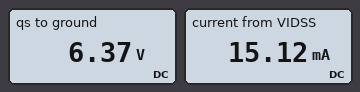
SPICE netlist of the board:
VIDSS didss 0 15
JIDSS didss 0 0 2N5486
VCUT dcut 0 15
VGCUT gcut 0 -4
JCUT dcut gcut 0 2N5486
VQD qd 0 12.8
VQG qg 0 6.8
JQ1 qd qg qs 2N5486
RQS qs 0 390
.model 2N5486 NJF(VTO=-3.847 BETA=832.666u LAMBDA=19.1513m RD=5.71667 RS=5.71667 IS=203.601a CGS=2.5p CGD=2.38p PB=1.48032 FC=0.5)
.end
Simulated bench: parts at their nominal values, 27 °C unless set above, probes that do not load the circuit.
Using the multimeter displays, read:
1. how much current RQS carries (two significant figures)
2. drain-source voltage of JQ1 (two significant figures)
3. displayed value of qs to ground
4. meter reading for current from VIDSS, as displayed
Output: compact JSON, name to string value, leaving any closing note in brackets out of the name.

{"how much current RQS carries": "16 mA", "drain-source voltage of JQ1": "6.4 V", "displayed value of qs to ground": "6.37 V", "meter reading for current from VIDSS, as displayed": "15.12 mA"}
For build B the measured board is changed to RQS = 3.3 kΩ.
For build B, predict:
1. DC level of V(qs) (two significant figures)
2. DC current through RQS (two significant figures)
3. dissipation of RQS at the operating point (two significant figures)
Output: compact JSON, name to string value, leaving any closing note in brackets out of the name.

{"DC level of V(qs)": "8.9 V", "DC current through RQS": "2.7 mA", "dissipation of RQS at the operating point": "24 mW"}
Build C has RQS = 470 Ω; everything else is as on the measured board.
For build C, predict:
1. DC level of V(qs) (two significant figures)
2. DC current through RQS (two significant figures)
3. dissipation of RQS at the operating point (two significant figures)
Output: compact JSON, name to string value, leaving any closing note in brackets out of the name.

{"DC level of V(qs)": "6.7 V", "DC current through RQS": "14 mA", "dissipation of RQS at the operating point": "94 mW"}
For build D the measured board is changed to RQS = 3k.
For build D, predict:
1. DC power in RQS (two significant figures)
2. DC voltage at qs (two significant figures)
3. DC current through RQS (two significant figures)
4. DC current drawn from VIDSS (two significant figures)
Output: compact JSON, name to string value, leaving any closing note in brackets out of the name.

{"DC power in RQS": "26 mW", "DC voltage at qs": "8.8 V", "DC current through RQS": "2.9 mA", "DC current drawn from VIDSS": "15 mA"}
